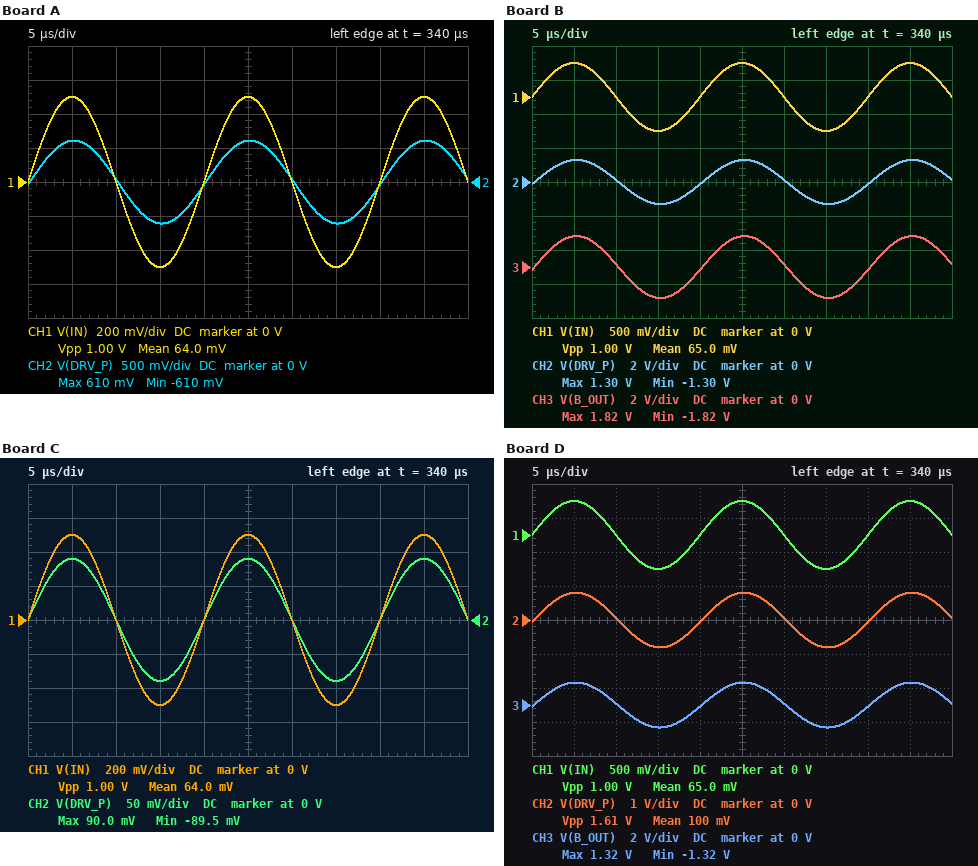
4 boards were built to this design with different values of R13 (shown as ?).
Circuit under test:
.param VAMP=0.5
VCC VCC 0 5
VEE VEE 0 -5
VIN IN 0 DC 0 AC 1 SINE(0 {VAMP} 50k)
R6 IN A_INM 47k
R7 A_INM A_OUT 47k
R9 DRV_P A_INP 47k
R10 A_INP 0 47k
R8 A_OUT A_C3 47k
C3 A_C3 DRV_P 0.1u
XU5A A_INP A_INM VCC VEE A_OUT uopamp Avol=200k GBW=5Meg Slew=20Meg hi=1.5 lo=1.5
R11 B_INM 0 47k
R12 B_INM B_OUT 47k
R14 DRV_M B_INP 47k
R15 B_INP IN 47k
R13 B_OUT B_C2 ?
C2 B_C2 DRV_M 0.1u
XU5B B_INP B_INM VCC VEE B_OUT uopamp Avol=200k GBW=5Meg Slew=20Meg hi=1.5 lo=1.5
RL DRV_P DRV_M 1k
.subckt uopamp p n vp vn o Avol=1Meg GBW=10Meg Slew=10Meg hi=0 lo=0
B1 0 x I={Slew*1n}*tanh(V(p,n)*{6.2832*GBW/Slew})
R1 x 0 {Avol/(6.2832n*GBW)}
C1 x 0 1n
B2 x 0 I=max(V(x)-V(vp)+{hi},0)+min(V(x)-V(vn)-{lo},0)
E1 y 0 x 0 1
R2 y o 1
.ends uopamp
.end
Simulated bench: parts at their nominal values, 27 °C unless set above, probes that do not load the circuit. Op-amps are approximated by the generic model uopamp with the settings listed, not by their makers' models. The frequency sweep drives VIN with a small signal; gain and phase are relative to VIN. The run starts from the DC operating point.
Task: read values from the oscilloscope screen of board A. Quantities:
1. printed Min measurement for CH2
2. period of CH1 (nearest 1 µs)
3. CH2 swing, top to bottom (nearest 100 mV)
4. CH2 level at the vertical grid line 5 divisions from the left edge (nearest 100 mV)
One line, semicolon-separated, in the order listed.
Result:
-610 mV; 20 µs; 1.2 V; 600 mV
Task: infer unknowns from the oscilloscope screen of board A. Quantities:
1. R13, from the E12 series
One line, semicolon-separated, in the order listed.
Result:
27 kΩ
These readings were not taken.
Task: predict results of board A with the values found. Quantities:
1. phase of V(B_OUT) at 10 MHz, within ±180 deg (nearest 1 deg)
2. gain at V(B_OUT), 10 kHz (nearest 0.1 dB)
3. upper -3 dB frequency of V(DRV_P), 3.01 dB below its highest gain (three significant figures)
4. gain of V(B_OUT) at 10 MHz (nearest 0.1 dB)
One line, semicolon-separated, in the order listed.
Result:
-80 deg; 7.1 dB; 671 kHz; -11.1 dB
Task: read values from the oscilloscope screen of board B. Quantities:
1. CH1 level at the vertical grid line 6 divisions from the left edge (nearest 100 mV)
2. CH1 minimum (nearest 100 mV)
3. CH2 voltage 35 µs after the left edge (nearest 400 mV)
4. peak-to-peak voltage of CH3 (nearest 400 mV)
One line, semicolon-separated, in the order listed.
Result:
0 V; -500 mV; -1.2 V; 3.6 V
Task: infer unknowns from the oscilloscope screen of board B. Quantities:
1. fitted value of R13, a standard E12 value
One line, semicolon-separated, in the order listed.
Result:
15 kΩ
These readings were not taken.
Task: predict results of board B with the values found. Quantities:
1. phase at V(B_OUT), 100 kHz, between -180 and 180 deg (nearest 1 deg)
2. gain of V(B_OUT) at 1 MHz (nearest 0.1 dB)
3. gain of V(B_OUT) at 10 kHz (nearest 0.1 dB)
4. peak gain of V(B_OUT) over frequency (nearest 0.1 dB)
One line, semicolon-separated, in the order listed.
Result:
-10 deg; 4.9 dB; 11.3 dB; 11.3 dB
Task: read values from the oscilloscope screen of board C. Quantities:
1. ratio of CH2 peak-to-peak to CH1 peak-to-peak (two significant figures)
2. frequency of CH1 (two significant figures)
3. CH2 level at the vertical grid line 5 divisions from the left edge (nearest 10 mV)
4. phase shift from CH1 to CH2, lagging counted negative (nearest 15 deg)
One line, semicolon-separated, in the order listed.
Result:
0.18; 50 kHz; 90 mV; 0 deg
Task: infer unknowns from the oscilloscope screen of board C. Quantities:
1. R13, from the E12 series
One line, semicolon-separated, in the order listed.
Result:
68 kΩ
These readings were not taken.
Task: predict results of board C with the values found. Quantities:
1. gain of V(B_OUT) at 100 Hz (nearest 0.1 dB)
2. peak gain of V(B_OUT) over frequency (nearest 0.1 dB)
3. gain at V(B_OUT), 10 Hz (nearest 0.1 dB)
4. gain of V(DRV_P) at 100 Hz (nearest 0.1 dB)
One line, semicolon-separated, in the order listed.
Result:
2.1 dB; 3.8 dB; 3.7 dB; -10.7 dB
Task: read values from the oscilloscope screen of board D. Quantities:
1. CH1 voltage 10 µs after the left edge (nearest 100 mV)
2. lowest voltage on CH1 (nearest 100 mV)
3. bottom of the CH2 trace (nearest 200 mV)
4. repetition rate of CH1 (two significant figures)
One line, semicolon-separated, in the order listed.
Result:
0 V; -500 mV; -800 mV; 50 kHz
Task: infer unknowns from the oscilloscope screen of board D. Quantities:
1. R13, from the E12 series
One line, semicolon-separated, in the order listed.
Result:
22 kΩ
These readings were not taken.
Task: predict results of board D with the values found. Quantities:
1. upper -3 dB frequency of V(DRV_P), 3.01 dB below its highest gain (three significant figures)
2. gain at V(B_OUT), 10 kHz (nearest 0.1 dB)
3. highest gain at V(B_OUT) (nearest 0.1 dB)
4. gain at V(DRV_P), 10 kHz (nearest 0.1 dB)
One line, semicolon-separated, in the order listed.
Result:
604 kHz; 8.5 dB; 8.5 dB; 4.2 dB
